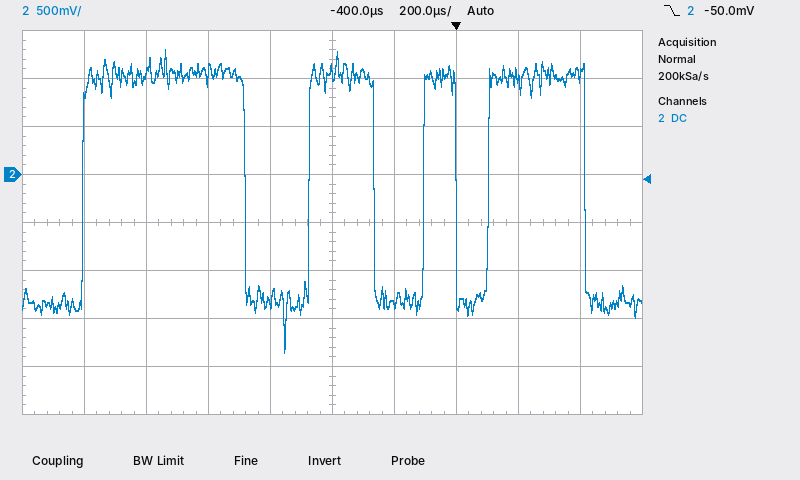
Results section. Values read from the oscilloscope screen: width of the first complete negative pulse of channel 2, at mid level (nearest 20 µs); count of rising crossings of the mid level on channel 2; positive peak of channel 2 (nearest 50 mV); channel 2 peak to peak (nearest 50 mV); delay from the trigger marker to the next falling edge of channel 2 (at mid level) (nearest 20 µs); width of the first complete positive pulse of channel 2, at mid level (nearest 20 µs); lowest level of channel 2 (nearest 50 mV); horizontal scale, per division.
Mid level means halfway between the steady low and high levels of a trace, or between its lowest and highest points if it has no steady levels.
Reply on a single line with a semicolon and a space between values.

200 µs; 4; 1.30 V; 3.15 V; 420 µs; 520 µs; -1.85 V; 200 µs
